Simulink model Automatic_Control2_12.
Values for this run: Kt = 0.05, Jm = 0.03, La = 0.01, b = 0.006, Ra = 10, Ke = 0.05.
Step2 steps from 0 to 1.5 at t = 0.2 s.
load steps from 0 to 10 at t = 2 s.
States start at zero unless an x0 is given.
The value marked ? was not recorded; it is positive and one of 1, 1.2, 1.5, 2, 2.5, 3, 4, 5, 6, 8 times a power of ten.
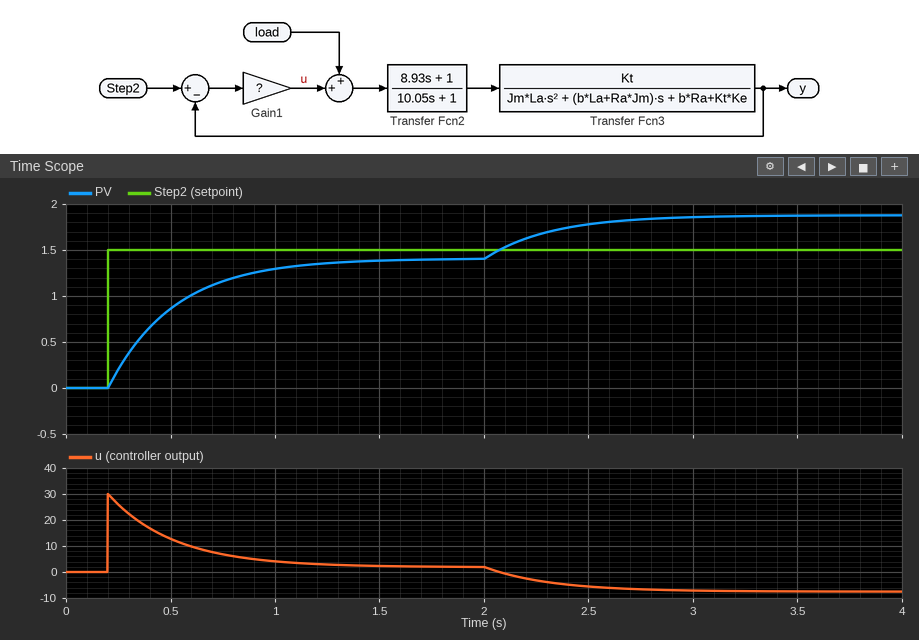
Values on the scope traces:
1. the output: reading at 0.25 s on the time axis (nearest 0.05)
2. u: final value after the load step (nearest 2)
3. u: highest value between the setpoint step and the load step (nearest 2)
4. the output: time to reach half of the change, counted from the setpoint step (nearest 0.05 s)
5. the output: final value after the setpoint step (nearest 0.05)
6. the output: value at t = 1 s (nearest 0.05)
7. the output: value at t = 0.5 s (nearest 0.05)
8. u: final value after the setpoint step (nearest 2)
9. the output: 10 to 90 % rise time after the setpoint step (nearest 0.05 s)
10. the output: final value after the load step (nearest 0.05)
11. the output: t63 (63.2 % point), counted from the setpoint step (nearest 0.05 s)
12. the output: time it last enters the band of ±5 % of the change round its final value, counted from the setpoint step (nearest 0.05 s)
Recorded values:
0.20
-8
30
0.20 s
1.40
1.30
0.85
2
0.70 s
1.90
0.30 s
0.95 s
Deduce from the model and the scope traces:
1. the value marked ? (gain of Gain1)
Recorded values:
20
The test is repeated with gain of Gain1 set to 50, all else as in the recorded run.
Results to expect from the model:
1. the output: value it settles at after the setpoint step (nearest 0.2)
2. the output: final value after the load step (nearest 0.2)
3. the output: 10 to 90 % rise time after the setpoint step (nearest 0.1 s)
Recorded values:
1.4
1.6
0.3 s
